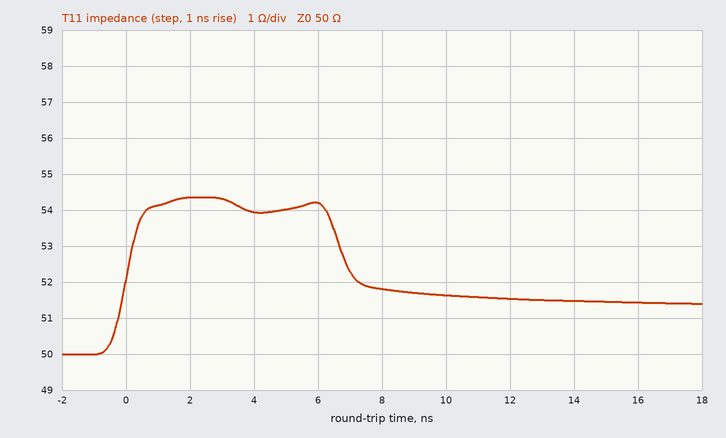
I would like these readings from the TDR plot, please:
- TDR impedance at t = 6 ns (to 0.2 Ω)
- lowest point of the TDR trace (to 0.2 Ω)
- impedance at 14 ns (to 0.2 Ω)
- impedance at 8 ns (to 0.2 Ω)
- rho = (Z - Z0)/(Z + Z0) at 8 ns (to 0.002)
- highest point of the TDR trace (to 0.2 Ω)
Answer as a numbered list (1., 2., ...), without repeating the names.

1. 54.2 Ω
2. 50.0 Ω
3. 51.4 Ω
4. 51.8 Ω
5. +0.018
6. 54.4 Ω
